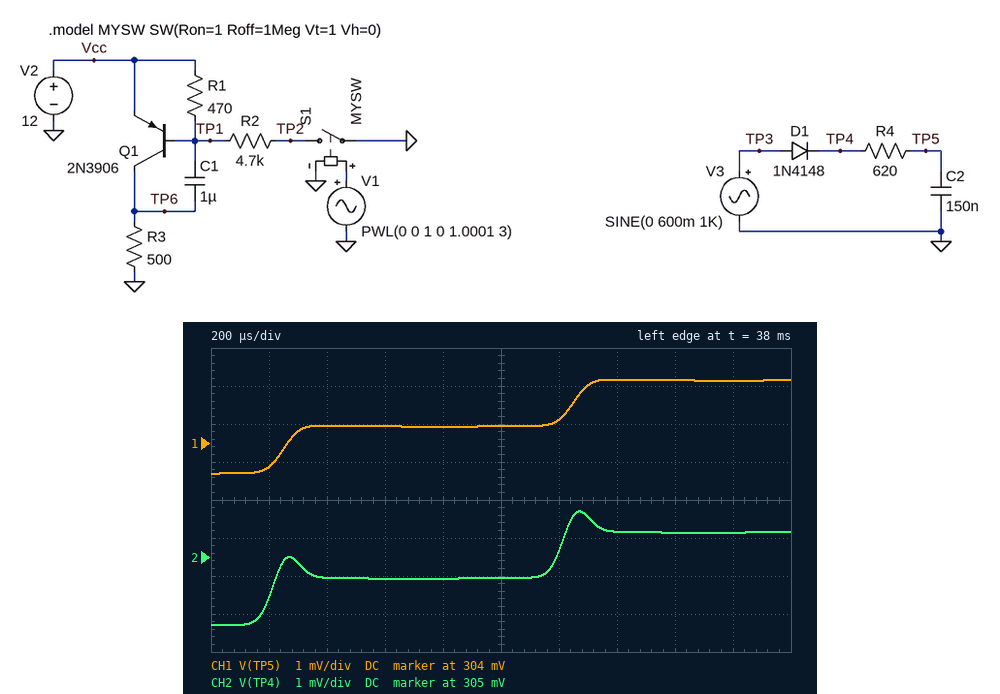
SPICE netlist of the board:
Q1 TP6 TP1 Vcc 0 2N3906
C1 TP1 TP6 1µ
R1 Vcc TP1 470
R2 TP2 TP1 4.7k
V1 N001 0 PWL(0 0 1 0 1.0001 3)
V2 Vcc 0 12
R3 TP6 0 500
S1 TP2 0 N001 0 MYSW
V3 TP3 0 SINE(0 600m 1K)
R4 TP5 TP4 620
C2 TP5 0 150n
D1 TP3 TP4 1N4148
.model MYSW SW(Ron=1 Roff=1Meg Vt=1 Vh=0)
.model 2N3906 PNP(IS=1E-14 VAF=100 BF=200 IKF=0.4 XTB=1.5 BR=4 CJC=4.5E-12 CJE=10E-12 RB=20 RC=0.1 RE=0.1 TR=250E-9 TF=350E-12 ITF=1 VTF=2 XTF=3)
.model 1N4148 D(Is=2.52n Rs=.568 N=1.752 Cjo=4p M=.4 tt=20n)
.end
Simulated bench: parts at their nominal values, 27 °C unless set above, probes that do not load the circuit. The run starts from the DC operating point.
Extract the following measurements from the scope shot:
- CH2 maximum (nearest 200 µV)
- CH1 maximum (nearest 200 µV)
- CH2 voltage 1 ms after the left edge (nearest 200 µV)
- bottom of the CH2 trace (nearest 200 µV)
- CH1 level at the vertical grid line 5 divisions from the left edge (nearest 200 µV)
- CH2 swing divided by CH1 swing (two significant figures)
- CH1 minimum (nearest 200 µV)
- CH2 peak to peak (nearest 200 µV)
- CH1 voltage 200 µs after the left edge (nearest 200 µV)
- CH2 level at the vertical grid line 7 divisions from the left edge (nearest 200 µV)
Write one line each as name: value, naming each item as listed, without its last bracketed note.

CH2 maximum: 306.2 mV
CH1 maximum: 305.6 mV
CH2 voltage 1 ms after the left edge: 304.4 mV
bottom of the CH2 trace: 303.2 mV
CH1 level at the vertical grid line 5 divisions from the left edge: 304.4 mV
CH2 swing divided by CH1 swing: 1.2
CH1 minimum: 303.2 mV
CH2 peak to peak: 3.0 mV
CH1 voltage 200 µs after the left edge: 303.4 mV
CH2 level at the vertical grid line 7 divisions from the left edge: 305.6 mV
